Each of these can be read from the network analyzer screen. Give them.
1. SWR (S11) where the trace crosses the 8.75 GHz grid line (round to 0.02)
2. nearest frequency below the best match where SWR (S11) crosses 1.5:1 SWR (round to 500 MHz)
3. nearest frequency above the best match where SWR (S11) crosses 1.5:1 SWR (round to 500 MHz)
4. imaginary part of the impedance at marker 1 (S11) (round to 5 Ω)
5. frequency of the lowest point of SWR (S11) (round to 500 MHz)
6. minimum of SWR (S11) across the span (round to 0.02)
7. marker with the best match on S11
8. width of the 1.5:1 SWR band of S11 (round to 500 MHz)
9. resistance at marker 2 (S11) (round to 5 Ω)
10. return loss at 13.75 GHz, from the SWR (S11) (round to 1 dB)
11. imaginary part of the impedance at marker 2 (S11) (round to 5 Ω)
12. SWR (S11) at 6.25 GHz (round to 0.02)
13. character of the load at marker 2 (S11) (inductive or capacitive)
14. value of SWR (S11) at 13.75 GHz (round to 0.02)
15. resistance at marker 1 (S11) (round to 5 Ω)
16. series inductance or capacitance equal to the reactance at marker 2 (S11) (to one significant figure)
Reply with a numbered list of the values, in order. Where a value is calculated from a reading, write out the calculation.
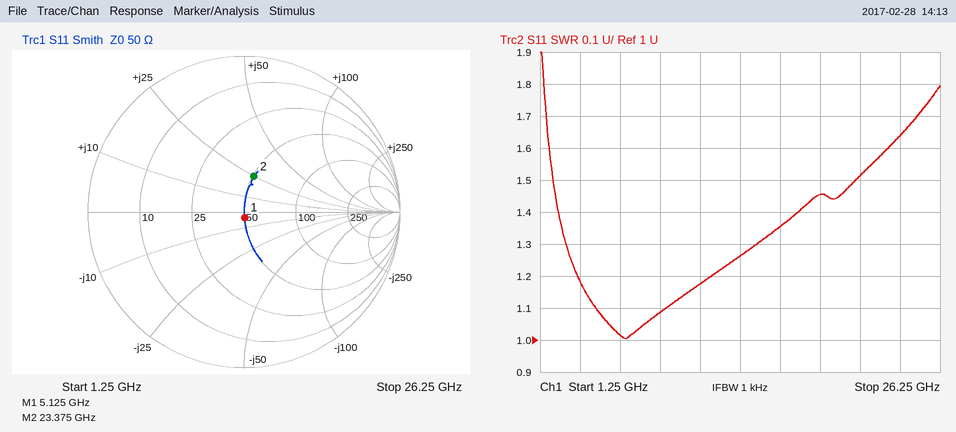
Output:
1. 1.08
2. 2.0 GHz
3. 21.0 GHz
4. -5 Ω
5. 6.5 GHz
6. 1.00
7. marker 1
8. 21.0 GHz − 2.0 GHz = 19.0 GHz
9. 50 Ω
10. −20 log10((1.26 − 1)/(1.26 + 1)) ≈ 19 dB
11. +25 Ω
12. 1.02
13. inductive
14. 1.26
15. 50 Ω
16. L = 25 Ω/(2π × 23.375 GHz) ≈ 170 pH, so 200 pH to one significant figure
